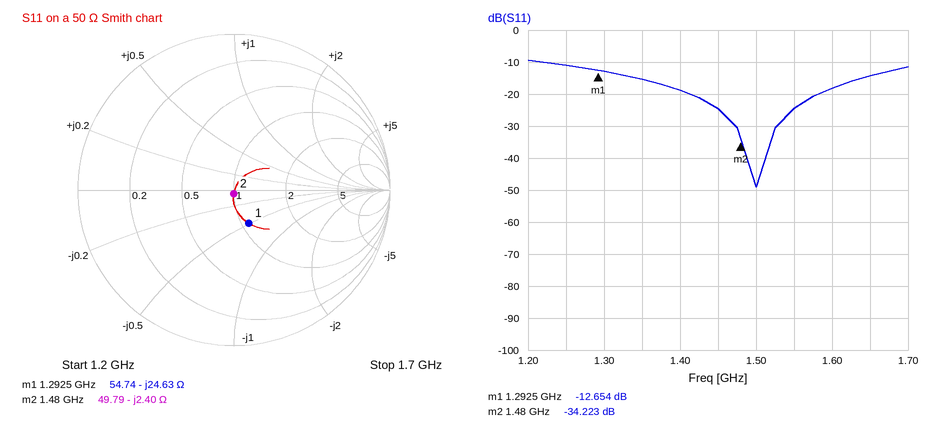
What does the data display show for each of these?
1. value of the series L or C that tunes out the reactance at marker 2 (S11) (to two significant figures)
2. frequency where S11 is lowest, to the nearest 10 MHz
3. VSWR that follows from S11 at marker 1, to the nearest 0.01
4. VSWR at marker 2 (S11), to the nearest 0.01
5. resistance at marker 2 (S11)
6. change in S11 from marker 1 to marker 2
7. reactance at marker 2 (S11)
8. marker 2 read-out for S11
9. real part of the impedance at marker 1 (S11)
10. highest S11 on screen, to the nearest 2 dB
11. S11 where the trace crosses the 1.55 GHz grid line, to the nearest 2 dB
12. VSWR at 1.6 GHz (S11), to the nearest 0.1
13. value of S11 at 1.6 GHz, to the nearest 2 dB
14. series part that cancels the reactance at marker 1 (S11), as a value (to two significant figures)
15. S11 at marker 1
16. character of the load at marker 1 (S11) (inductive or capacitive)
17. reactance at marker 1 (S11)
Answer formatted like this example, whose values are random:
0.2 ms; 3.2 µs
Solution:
260 pH; 1.50 GHz; 1.61; 1.04; 49.79 Ω; -21.569 dB; -2.40 Ω; -34.223 dB; 54.74 Ω; -10 dB; -24 dB; 1.3; -18 dB; 3.0 nH; -12.654 dB; capacitive; -24.63 Ω
